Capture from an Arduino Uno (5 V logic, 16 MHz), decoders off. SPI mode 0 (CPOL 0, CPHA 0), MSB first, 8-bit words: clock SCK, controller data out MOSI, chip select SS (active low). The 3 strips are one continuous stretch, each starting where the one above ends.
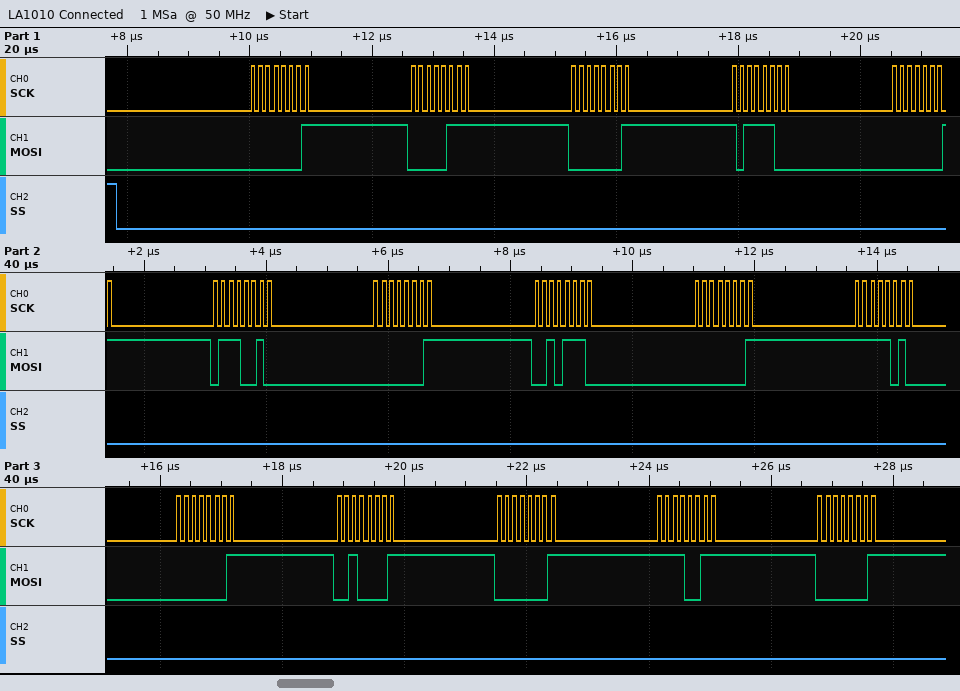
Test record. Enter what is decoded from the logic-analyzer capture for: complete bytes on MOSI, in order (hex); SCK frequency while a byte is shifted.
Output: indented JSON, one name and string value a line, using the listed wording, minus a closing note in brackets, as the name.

{
  "complete bytes on MOSI, in order": "01 07 01 BC 01 72 01 2E 01 FA 01 21 01 F3 01",
  "SCK frequency while a byte is shifted": "8 MHz"
}
